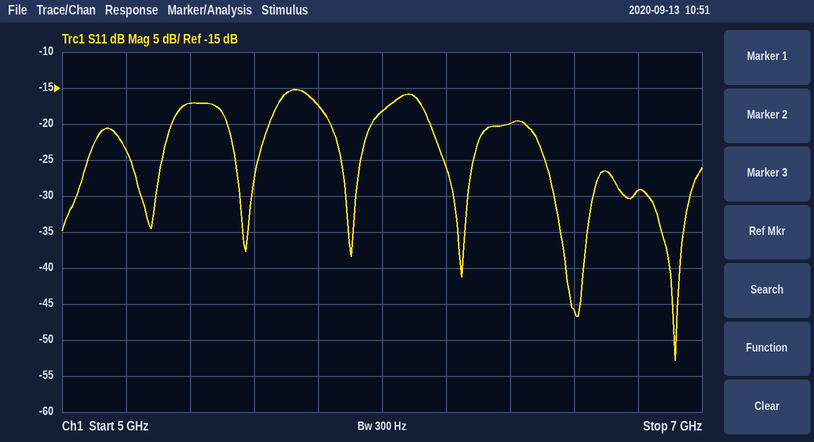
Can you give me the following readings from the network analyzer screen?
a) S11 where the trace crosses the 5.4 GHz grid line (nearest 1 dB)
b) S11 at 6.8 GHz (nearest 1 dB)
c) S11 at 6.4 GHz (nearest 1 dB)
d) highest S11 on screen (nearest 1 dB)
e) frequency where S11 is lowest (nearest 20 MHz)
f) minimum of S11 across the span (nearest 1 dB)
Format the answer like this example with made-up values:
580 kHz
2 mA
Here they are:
-17 dB
-29 dB
-20 dB
-15 dB
6.92 GHz
-53 dB
